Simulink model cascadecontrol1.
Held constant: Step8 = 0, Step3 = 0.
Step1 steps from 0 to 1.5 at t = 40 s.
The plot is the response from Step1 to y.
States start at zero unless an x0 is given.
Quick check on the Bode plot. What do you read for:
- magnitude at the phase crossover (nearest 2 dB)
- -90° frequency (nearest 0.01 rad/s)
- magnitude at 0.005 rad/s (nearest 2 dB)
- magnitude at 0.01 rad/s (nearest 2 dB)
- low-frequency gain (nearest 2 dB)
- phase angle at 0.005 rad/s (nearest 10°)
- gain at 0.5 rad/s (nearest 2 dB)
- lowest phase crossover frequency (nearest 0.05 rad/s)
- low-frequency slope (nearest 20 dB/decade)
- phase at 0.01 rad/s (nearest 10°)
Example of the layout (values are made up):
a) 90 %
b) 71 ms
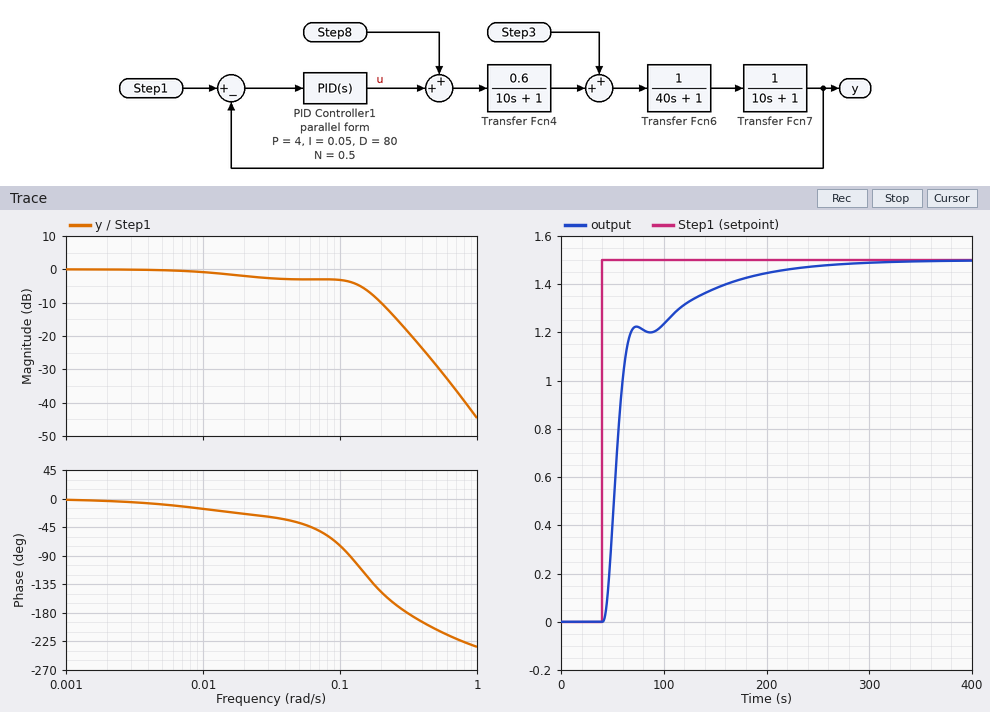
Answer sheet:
a) -18 dB
b) 0.12 rad/s
c) 0 dB
d) 0 dB
e) 0 dB
f) -10°
g) -28 dB
h) 0.30 rad/s
i) 0 dB/decade
j) -20°
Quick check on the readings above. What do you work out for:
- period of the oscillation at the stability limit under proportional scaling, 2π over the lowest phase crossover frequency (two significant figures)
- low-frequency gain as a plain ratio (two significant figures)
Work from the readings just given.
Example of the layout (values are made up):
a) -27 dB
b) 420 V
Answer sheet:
a) 21 s
b) 1.0
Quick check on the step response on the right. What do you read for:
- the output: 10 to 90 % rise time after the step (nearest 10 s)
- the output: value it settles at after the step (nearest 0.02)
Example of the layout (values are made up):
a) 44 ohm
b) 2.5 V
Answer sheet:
a) 90 s
b) 1.50
